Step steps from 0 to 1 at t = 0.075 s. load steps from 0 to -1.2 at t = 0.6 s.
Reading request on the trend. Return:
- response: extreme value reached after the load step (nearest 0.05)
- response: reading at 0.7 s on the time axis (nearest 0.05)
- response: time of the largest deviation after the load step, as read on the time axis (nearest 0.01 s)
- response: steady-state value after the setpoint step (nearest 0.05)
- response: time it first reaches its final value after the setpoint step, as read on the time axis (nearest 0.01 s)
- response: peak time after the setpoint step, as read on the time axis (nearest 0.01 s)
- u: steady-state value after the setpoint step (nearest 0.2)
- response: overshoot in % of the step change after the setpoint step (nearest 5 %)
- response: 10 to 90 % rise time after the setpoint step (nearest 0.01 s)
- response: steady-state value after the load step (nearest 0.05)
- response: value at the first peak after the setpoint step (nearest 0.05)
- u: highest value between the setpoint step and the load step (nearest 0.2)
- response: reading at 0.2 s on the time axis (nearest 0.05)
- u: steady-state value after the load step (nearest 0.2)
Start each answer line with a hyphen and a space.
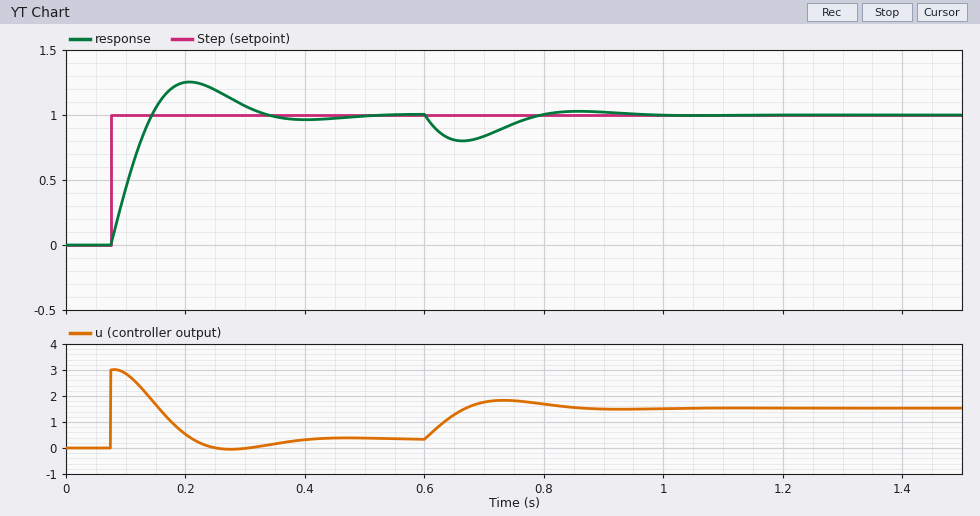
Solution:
- 0.80
- 0.85
- 0.66 s
- 1.00
- 0.14 s
- 0.21 s
- 0.4
- 25 %
- 0.05 s
- 1.00
- 1.25
- 3.0
- 1.25
- 1.6
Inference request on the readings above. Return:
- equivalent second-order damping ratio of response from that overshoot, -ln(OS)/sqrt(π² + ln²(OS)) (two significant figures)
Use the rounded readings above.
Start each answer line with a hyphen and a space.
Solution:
- 0.40
